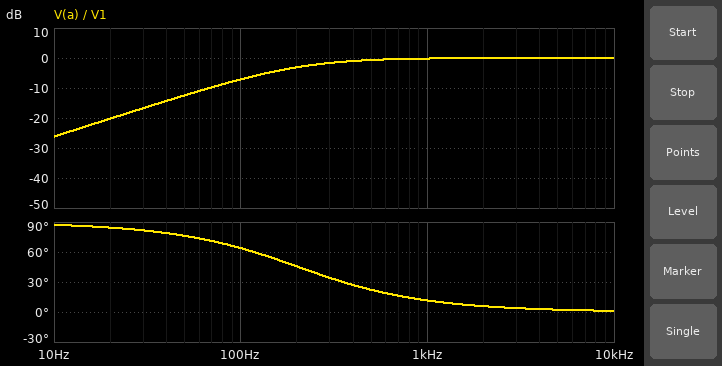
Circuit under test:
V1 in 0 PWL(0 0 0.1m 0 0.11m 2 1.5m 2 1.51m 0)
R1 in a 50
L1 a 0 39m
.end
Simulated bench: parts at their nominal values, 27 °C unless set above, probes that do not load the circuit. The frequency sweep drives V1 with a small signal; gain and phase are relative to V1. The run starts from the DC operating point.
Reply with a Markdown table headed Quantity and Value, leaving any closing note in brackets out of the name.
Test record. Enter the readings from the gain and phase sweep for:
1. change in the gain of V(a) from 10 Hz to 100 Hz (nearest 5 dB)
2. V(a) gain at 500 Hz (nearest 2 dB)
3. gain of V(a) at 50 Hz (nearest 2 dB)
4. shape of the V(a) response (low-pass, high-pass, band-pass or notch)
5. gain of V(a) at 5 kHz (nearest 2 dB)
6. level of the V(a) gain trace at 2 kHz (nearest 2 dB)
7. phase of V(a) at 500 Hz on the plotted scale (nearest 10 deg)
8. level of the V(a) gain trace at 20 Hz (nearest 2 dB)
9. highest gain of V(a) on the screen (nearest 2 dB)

| Quantity | Value |
|---|---|
| change in the gain of V(a) from 10 Hz to 100 Hz | 20 dB |
| V(a) gain at 500 Hz | 0 dB |
| gain of V(a) at 50 Hz | -12 dB |
| shape of the V(a) response | high-pass |
| gain of V(a) at 5 kHz | 0 dB |
| level of the V(a) gain trace at 2 kHz | 0 dB |
| phase of V(a) at 500 Hz on the plotted scale | 20 deg |
| level of the V(a) gain trace at 20 Hz | -20 dB |
| highest gain of V(a) on the screen | 0 dB |
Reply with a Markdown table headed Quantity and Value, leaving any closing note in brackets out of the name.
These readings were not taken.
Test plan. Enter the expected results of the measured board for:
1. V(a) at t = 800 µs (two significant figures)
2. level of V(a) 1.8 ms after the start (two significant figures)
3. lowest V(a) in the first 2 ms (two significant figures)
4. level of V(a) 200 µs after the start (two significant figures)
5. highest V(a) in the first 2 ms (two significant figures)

| Quantity | Value |
|---|---|
| V(a) at t = 800 µs | 820 mV |
| level of V(a) 1.8 ms after the start | -1.1 V |
| lowest V(a) in the first 2 ms | -1.7 V |
| level of V(a) 200 µs after the start | 1.8 V |
| highest V(a) in the first 2 ms | 2.0 V |
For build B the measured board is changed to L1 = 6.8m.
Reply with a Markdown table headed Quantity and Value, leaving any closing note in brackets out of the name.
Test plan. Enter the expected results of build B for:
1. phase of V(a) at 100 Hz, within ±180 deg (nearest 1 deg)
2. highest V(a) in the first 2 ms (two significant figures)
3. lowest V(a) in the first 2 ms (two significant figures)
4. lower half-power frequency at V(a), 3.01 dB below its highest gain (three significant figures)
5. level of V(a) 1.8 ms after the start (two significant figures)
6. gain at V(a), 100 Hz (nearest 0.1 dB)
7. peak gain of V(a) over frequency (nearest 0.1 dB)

| Quantity | Value |
|---|---|
| phase of V(a) at 100 Hz, within ±180 deg | 85 deg |
| highest V(a) in the first 2 ms | 1.9 V |
| lowest V(a) in the first 2 ms | -1.9 V |
| lower half-power frequency at V(a), 3.01 dB below its highest gain | 1.17 kHz |
| level of V(a) 1.8 ms after the start | -230 mV |
| gain at V(a), 100 Hz | -21.4 dB |
| peak gain of V(a) over frequency | 0 dB |
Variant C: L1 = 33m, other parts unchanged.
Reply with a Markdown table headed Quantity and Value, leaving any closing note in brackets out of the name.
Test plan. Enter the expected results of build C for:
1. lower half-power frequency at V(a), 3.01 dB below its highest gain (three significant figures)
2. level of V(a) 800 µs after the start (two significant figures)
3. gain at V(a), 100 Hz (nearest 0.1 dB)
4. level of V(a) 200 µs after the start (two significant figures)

| Quantity | Value |
|---|---|
| lower half-power frequency at V(a), 3.01 dB below its highest gain | 241 Hz |
| level of V(a) 800 µs after the start | 700 mV |
| gain at V(a), 100 Hz | -8.3 dB |
| level of V(a) 200 µs after the start | 1.7 V |
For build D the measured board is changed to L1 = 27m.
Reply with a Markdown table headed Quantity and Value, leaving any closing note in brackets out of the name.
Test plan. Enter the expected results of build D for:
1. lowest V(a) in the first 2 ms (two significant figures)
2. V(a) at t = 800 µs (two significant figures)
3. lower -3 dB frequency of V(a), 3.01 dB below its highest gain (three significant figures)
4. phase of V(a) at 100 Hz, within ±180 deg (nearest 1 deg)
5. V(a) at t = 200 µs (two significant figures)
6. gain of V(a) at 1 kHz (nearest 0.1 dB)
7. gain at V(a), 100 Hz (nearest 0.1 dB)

| Quantity | Value |
|---|---|
| lowest V(a) in the first 2 ms | -1.8 V |
| V(a) at t = 800 µs | 550 mV |
| lower -3 dB frequency of V(a), 3.01 dB below its highest gain | 295 Hz |
| phase of V(a) at 100 Hz, within ±180 deg | 71 deg |
| V(a) at t = 200 µs | 1.7 V |
| gain of V(a) at 1 kHz | -0.4 dB |
| gain at V(a), 100 Hz | -9.9 dB |
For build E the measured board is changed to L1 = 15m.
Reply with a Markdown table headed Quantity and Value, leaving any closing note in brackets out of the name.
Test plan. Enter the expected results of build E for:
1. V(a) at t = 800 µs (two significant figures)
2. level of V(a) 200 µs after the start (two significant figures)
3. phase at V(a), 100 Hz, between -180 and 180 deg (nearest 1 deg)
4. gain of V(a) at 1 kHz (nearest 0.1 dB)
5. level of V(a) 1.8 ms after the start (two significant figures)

| Quantity | Value |
|---|---|
| V(a) at t = 800 µs | 200 mV |
| level of V(a) 200 µs after the start | 1.5 V |
| phase at V(a), 100 Hz, between -180 and 180 deg | 79 deg |
| gain of V(a) at 1 kHz | -1.1 dB |
| level of V(a) 1.8 ms after the start | -740 mV |
